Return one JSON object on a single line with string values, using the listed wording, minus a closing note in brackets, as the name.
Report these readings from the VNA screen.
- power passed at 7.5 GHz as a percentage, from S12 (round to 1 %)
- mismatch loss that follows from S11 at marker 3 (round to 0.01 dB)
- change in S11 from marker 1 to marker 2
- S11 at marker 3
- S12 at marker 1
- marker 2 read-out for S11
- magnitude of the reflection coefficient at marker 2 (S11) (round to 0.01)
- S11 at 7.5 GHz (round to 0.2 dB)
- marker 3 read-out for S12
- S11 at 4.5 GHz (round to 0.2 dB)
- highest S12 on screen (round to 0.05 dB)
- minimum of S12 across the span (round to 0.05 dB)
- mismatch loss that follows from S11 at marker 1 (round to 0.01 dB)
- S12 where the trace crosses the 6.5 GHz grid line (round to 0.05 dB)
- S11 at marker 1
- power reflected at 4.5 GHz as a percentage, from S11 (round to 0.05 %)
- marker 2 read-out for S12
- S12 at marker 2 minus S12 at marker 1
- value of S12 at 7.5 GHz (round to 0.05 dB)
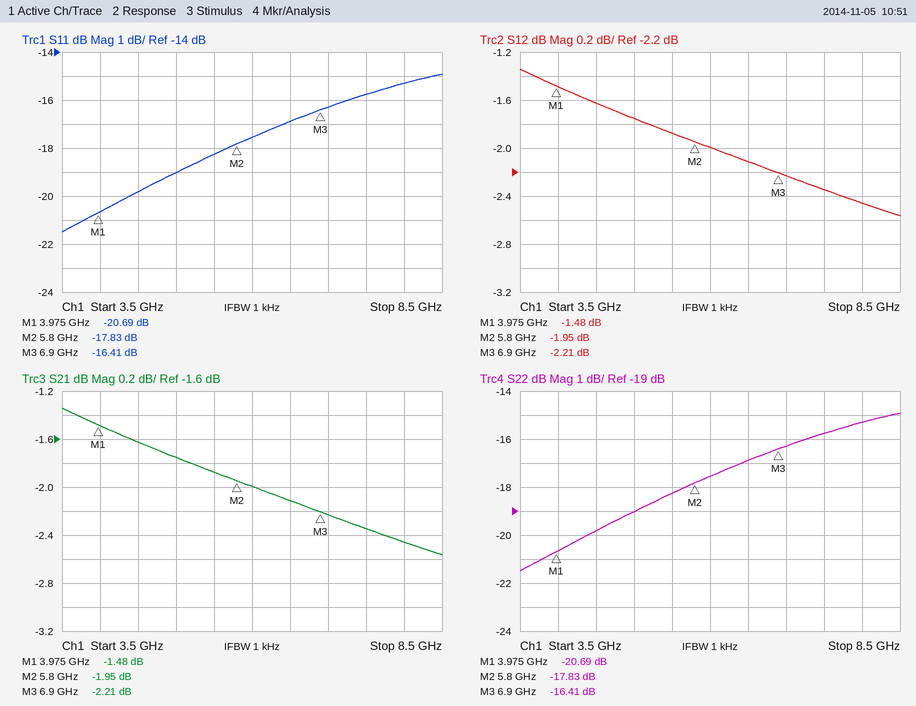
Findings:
{"power passed at 7.5 GHz as a percentage, from S12": "58 %", "mismatch loss that follows from S11 at marker 3": "0.10 dB", "change in S11 from marker 1 to marker 2": "2.86 dB", "S11 at marker 3": "-16.41 dB", "S12 at marker 1": "-1.48 dB", "marker 2 read-out for S11": "-17.83 dB", "magnitude of the reflection coefficient at marker 2 (S11)": "0.13", "S11 at 7.5 GHz": "-15.8 dB", "marker 3 read-out for S12": "-2.21 dB", "S11 at 4.5 GHz": "-19.8 dB", "highest S12 on screen": "-1.35 dB", "minimum of S12 across the span": "-2.55 dB", "mismatch loss that follows from S11 at marker 1": "0.04 dB", "S12 where the trace crosses the 6.5 GHz grid line": "-2.10 dB", "S11 at marker 1": "-20.69 dB", "power reflected at 4.5 GHz as a percentage, from S11": "1.05 %", "marker 2 read-out for S12": "-1.95 dB", "S12 at marker 2 minus S12 at marker 1": "-0.47 dB", "value of S12 at 7.5 GHz": "-2.35 dB"}
